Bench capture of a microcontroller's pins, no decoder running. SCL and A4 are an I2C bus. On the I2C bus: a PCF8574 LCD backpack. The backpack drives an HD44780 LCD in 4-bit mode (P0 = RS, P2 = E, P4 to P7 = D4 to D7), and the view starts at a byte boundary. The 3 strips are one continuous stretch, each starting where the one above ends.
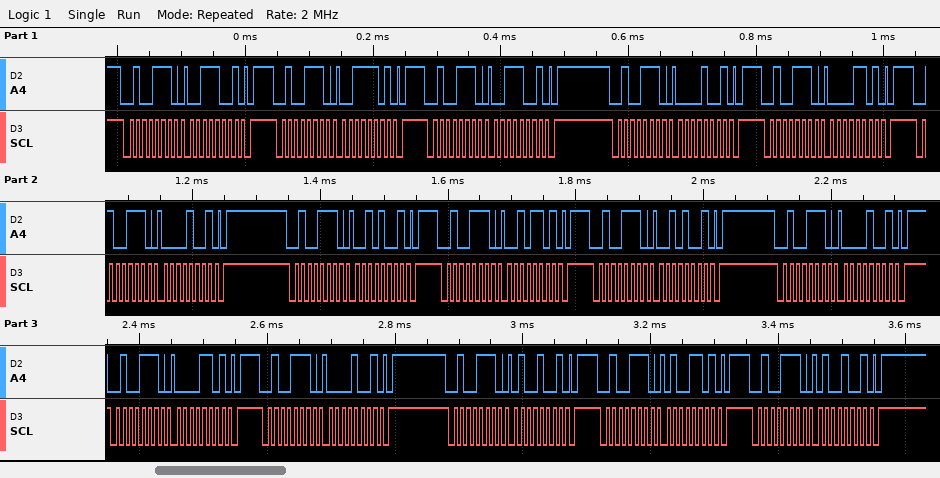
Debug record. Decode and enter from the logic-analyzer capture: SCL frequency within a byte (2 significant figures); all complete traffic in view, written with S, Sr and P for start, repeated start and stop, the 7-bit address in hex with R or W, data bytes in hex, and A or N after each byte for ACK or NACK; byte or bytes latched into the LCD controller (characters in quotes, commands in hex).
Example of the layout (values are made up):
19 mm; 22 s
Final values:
100 kHz; S 27W A 39 A P S 27W A 3D A P S 27W A 39 A P S 27W A 09 A P S 27W A 0D A P S 27W A 09 A P S 27W A 29 A P S 27W A 2D A P S 27W A 29 A P S 27W A 09 A P S 27W A 0D A P S 27W A 09 A P S 27W A 49 A P S 27W A 4D A P S 27W A 49 A P; '0' ' '
